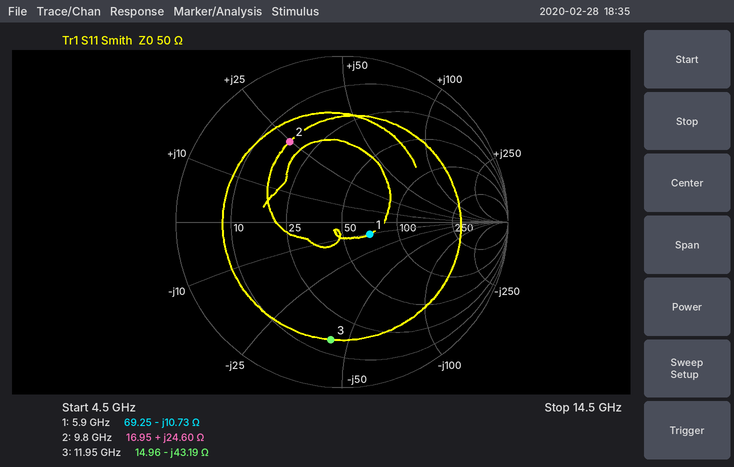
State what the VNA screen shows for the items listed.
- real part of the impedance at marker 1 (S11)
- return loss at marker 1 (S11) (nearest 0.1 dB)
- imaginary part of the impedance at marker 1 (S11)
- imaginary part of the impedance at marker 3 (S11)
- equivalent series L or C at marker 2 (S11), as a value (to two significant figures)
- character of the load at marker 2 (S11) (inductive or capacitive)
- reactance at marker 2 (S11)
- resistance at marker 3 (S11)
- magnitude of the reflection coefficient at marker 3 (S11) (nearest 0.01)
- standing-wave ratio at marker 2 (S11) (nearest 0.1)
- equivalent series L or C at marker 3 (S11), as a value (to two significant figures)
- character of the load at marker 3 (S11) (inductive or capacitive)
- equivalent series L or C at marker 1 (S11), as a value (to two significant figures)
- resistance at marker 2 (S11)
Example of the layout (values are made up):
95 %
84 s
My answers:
69.25 Ω
14.7 dB
-10.73 Ω
-43.19 Ω
400 pH
inductive
+24.60 Ω
14.96 Ω
0.71
3.7
310 fF
capacitive
2.5 pF
16.95 Ω
